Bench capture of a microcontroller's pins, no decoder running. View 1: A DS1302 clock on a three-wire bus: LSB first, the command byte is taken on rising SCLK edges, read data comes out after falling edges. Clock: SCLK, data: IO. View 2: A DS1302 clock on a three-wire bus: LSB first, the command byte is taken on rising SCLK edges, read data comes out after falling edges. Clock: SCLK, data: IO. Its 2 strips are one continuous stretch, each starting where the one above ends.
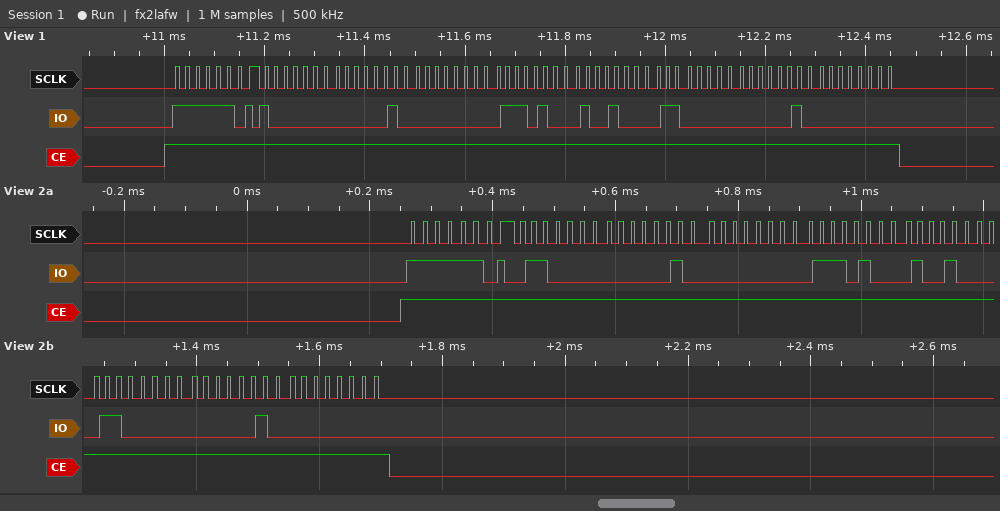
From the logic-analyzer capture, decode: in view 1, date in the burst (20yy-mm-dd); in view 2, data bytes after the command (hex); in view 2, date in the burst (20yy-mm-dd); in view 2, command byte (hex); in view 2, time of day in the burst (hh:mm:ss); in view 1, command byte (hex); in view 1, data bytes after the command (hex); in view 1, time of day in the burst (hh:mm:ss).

2020-09-17
06 20 00 17 09 03 20 00
2020-09-17
0xBF
00:20:06
0xBF
01 20 00 17 09 03 20 00
00:20:01
